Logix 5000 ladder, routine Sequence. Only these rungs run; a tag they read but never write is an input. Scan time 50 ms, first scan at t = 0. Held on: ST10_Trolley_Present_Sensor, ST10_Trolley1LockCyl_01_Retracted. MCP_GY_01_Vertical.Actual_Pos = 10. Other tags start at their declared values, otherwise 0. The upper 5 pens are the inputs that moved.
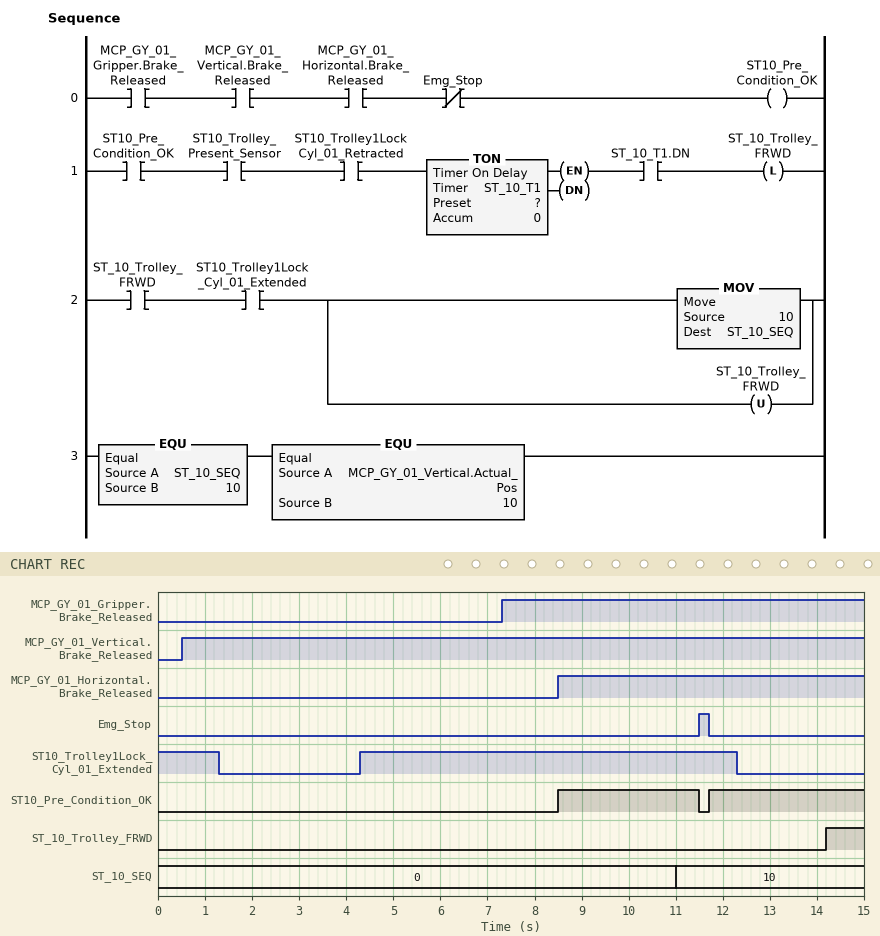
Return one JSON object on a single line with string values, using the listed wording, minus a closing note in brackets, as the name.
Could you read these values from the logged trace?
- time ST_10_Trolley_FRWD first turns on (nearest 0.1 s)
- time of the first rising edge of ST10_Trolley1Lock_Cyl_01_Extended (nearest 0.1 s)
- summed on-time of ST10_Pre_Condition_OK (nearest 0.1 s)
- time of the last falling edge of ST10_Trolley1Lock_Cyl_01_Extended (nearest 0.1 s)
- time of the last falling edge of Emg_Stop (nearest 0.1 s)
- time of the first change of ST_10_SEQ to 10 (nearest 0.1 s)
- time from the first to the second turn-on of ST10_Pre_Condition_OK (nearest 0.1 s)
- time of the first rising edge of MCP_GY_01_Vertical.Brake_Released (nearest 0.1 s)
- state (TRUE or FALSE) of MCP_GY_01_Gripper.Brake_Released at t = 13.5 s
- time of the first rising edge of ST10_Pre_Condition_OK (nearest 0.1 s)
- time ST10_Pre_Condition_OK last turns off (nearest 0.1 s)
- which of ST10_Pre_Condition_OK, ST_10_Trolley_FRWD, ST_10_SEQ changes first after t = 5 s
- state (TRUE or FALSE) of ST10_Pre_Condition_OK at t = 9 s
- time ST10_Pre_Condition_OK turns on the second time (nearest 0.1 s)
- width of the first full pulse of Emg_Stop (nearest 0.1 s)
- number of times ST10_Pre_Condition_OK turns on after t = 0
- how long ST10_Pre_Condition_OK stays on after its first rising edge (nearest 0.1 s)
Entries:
{"time ST_10_Trolley_FRWD first turns on": "14.2 s", "time of the first rising edge of ST10_Trolley1Lock_Cyl_01_Extended": "4.3 s", "summed on-time of ST10_Pre_Condition_OK": "6.3 s", "time of the last falling edge of ST10_Trolley1Lock_Cyl_01_Extended": "12.3 s", "time of the last falling edge of Emg_Stop": "11.7 s", "time of the first change of ST_10_SEQ to 10": "11.0 s", "time from the first to the second turn-on of ST10_Pre_Condition_OK": "3.2 s", "time of the first rising edge of MCP_GY_01_Vertical.Brake_Released": "0.5 s", "state (TRUE or FALSE) of MCP_GY_01_Gripper.Brake_Released at t = 13.5 s": "TRUE", "time of the first rising edge of ST10_Pre_Condition_OK": "8.5 s", "time ST10_Pre_Condition_OK last turns off": "11.5 s", "which of ST10_Pre_Condition_OK, ST_10_Trolley_FRWD, ST_10_SEQ changes first after t = 5 s": "ST10_Pre_Condition_OK", "state (TRUE or FALSE) of ST10_Pre_Condition_OK at t = 9 s": "TRUE", "time ST10_Pre_Condition_OK turns on the second time": "11.7 s", "width of the first full pulse of Emg_Stop": "0.2 s", "number of times ST10_Pre_Condition_OK turns on after t = 0": "2", "how long ST10_Pre_Condition_OK stays on after its first rising edge": "3.0 s"}
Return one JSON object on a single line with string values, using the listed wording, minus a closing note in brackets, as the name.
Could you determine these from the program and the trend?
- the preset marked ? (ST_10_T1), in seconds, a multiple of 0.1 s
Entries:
{"the preset marked ? (ST_10_T1), in seconds, a multiple of 0.1 s": "2.5 s"}
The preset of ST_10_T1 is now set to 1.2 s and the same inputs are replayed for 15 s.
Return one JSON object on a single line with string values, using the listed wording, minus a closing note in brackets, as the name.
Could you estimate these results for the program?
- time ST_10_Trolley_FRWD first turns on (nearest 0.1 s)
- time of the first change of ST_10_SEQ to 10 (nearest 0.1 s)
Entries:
{"time ST_10_Trolley_FRWD first turns on": "12.9 s", "time of the first change of ST_10_SEQ to 10": "9.7 s"}
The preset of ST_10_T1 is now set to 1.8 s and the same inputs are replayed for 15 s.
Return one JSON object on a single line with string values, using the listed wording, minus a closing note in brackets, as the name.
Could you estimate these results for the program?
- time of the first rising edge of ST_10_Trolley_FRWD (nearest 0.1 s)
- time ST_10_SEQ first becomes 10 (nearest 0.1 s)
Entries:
{"time of the first rising edge of ST_10_Trolley_FRWD": "13.5 s", "time ST_10_SEQ first becomes 10": "10.3 s"}
